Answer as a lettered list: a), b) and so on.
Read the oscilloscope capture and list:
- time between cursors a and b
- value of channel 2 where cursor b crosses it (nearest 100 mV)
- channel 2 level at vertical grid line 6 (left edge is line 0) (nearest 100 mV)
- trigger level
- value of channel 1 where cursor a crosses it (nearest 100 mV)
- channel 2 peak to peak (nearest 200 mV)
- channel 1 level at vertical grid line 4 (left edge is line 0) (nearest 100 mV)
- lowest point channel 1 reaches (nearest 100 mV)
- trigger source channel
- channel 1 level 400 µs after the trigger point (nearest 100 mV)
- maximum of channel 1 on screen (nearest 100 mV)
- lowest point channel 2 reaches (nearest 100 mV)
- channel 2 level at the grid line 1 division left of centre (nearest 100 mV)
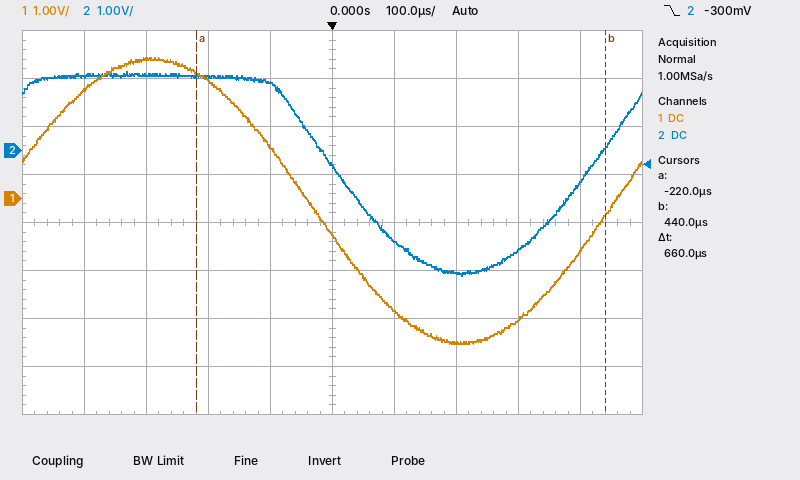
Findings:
a) 660 µs
b) 100 mV
c) -1.9 V
d) -300 mV
e) 2.6 V
f) 4.2 V
g) 1.1 V
h) -3.0 V
i) channel 2
j) -1.1 V
k) 2.9 V
l) -2.6 V
m) 1.4 V
